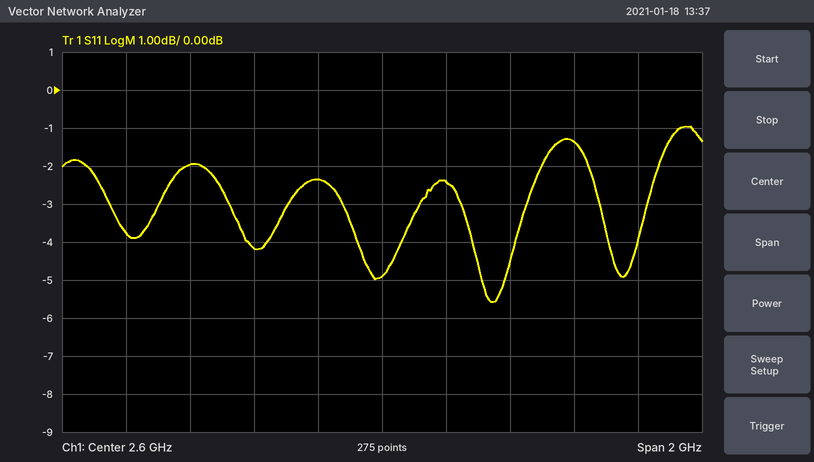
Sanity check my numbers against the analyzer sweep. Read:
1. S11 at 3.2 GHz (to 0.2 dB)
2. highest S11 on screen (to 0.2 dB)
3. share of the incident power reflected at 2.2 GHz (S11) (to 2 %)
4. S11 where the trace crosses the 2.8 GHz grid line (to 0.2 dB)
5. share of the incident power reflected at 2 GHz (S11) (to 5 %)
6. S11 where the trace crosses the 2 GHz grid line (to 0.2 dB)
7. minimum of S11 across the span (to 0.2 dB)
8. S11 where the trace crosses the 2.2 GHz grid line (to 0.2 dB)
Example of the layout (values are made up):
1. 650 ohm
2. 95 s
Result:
1. -1.4 dB
2. -1.0 dB
3. 38 %
4. -2.4 dB
5. 65 %
6. -2.0 dB
7. -5.6 dB
8. -4.2 dB
